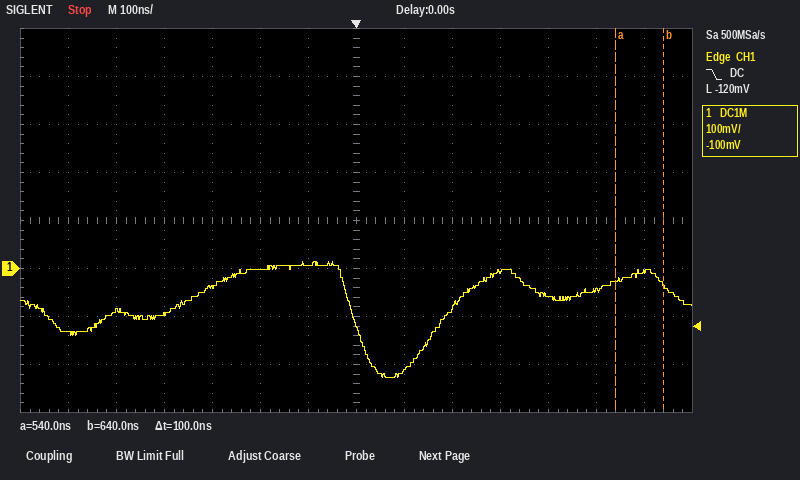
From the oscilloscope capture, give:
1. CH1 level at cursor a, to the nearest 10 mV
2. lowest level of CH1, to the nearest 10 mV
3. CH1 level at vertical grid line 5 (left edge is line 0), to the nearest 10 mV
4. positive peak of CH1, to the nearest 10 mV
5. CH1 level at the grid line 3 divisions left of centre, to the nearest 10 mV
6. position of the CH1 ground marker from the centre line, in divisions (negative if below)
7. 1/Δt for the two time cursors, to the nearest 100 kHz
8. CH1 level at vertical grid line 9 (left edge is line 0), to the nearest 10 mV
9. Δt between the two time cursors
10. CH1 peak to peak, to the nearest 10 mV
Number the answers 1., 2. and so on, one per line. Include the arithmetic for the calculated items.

1. -20 mV
2. -230 mV
3. 0 mV
4. 10 mV
5. -40 mV
6. -1.0 div
7. 1 / 100 ns ≈ 10.0 MHz
8. -80 mV
9. 100 ns
10. 10 mV − (-230 mV) = 240 mV
